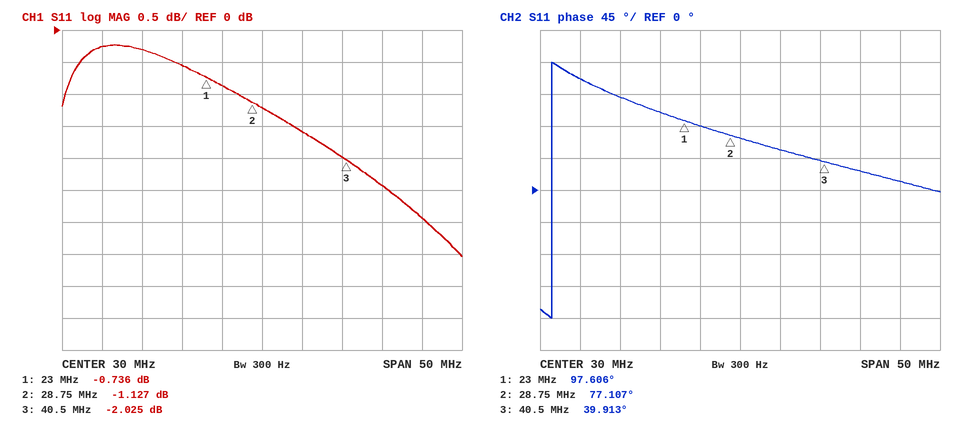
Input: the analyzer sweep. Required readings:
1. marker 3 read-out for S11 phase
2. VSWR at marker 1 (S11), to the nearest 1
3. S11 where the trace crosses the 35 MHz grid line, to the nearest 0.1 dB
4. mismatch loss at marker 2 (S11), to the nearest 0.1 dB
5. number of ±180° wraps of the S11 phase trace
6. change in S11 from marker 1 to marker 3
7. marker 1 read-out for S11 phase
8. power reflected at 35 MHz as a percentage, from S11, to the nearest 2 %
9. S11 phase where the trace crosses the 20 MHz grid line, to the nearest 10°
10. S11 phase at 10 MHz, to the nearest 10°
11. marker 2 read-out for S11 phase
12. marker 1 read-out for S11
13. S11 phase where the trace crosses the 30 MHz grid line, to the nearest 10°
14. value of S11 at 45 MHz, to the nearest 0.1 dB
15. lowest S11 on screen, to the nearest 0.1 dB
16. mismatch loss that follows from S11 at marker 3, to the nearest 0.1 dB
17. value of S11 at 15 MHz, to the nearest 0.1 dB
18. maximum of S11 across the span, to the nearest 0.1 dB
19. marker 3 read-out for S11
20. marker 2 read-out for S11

39.913°
24
-1.6 dB
6.4 dB
1
-1.289 dB
97.606°
70 %
110°
160°
77.107°
-0.736 dB
70°
-2.4 dB
-3.5 dB
4.3 dB
-0.3 dB
-0.2 dB
-2.025 dB
-1.127 dB
